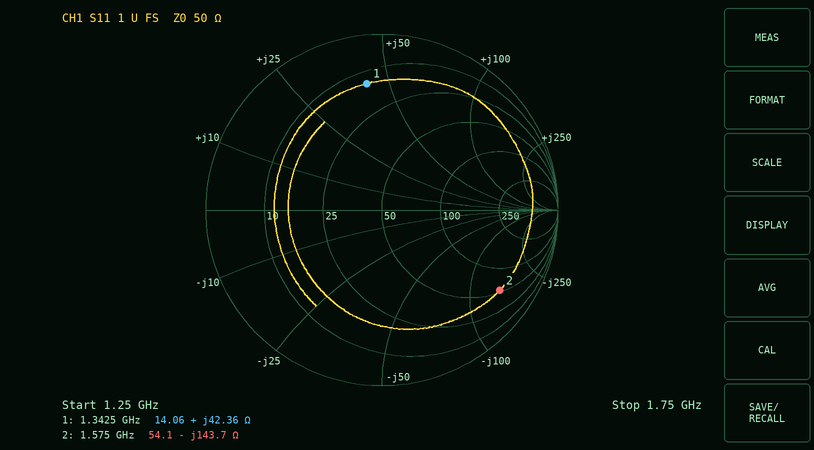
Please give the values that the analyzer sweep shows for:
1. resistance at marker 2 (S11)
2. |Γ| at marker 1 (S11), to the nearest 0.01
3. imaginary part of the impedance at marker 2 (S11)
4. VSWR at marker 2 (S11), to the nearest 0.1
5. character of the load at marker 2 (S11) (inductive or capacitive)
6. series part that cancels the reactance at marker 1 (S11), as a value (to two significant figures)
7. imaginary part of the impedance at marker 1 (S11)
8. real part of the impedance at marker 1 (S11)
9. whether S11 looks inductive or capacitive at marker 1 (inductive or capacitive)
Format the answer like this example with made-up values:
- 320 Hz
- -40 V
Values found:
- 54.1 Ω
- 0.72
- -143.7 Ω
- 9.5
- capacitive
- 2.8 pF
- +42.36 Ω
- 14.06 Ω
- inductive
